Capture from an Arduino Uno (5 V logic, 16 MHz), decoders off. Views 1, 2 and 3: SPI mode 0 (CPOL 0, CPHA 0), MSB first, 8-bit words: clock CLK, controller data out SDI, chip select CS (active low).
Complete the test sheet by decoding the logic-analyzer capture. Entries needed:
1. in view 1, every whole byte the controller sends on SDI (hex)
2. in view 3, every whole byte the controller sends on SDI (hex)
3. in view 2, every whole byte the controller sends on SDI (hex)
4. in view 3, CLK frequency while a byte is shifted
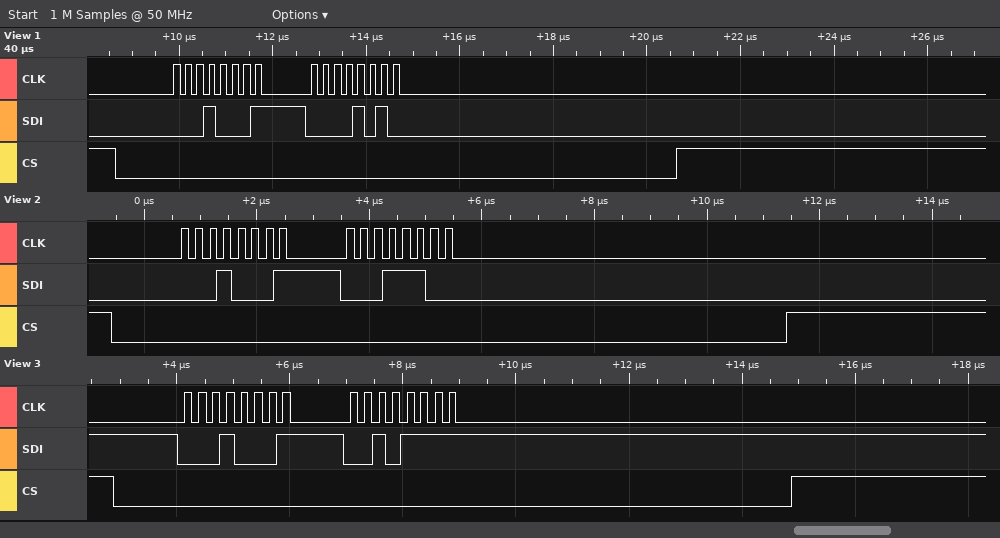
0x11 0x0A
11 2F
11 1C
4 MHz
